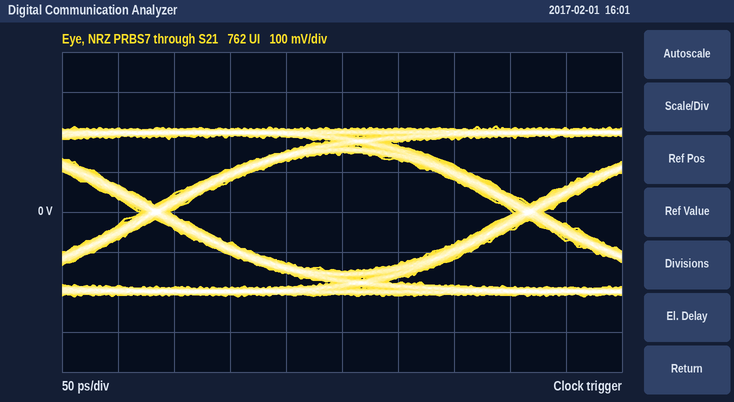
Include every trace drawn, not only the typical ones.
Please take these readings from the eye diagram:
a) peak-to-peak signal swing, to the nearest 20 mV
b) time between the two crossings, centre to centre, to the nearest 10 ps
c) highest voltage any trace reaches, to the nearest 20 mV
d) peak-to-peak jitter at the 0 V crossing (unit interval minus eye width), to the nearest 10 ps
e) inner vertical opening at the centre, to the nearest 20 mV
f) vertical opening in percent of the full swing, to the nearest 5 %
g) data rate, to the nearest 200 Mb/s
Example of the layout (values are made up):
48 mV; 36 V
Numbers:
420 mV; 330 ps; 220 mV; 30 ps; 300 mV; 70 %; 3.0 Gb/s
